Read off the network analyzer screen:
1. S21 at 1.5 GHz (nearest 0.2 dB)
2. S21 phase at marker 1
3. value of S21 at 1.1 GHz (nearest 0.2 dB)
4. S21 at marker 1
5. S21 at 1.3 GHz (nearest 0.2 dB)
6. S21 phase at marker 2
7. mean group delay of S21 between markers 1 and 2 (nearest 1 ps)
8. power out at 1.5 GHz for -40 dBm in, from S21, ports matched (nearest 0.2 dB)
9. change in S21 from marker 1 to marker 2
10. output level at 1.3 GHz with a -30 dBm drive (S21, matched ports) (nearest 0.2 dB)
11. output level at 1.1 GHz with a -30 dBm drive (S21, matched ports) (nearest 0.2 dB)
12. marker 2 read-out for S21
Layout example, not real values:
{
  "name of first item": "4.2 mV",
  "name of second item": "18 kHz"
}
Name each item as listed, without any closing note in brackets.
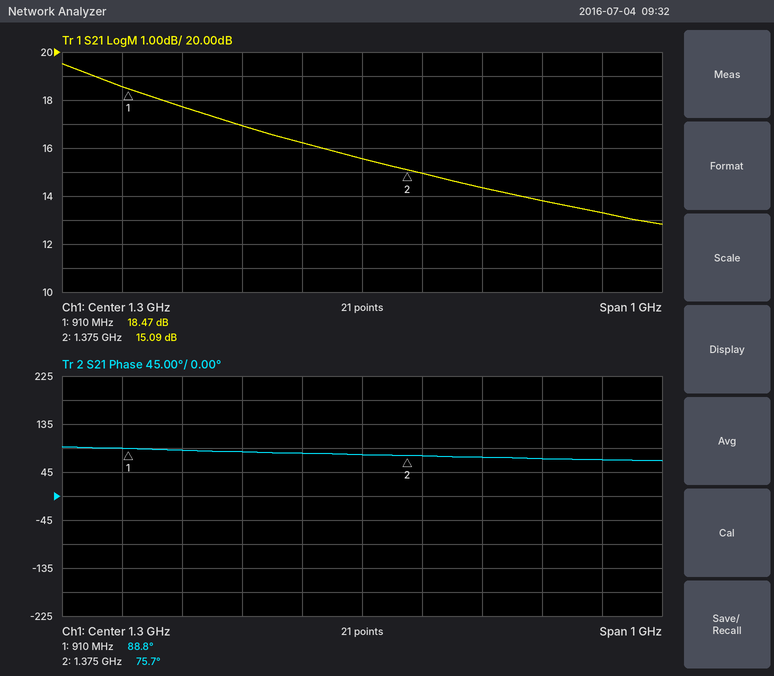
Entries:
{
  "S21 at 1.5 GHz": "14.4 dB",
  "S21 phase at marker 1": "88.8°",
  "value of S21 at 1.1 GHz": "17.0 dB",
  "S21 at marker 1": "18.47 dB",
  "S21 at 1.3 GHz": "15.6 dB",
  "S21 phase at marker 2": "75.7°",
  "mean group delay of S21 between markers 1 and 2": "78 ps",
  "power out at 1.5 GHz for -40 dBm in, from S21, ports matched": "-25.6 dBm",
  "change in S21 from marker 1 to marker 2": "-3.38 dB",
  "output level at 1.3 GHz with a -30 dBm drive (S21, matched ports)": "-14.4 dBm",
  "output level at 1.1 GHz with a -30 dBm drive (S21, matched ports)": "-13.0 dBm",
  "marker 2 read-out for S21": "15.09 dB"
}
